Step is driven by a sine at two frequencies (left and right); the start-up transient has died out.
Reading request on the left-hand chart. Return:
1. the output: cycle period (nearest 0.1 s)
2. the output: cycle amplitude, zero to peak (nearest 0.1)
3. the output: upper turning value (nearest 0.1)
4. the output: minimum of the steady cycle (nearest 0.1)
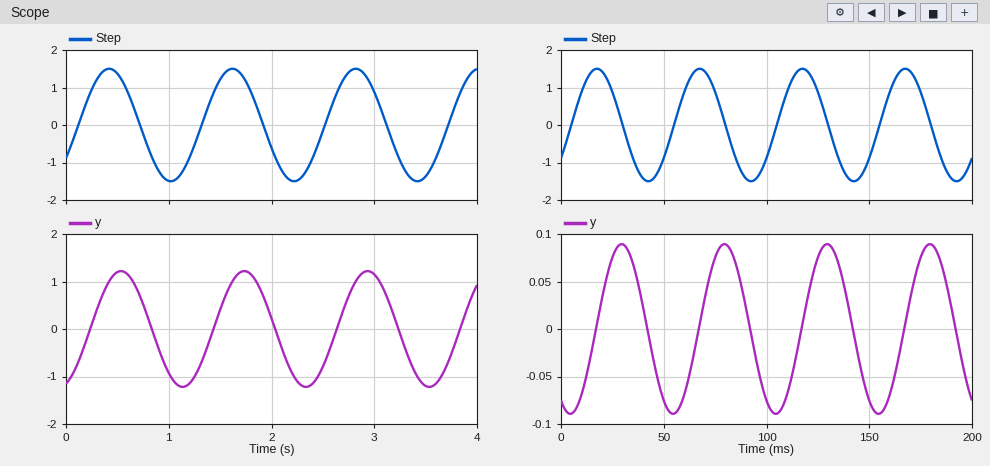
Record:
1.2 s
1.2
1.2
-1.2
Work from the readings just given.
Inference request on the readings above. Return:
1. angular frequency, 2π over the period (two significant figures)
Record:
5.2 rad/s
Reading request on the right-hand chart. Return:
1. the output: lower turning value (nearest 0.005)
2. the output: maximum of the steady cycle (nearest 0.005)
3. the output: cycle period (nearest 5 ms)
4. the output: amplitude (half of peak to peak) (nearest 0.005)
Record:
-0.090
0.090
50 ms
0.090
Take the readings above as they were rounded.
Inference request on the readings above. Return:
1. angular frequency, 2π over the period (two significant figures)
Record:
0.13 rad/ms
